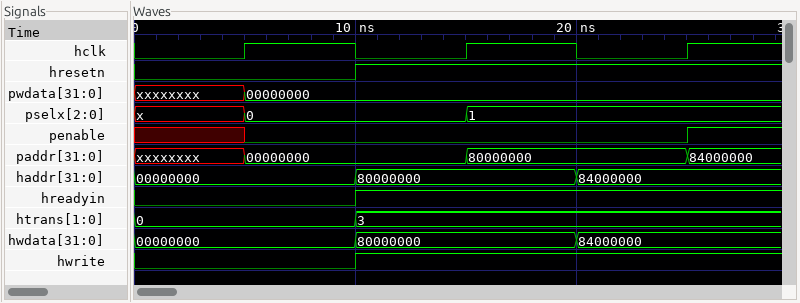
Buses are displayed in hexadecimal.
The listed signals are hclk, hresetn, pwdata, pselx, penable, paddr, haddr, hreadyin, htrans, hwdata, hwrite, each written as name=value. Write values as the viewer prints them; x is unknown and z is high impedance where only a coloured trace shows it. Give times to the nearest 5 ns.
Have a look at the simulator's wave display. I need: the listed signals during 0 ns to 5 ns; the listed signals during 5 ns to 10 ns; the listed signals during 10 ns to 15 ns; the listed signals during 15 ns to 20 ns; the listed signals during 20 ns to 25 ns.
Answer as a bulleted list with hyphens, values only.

- hclk=0, hresetn=0, pwdata=xxxxxxxx, pselx=x, penable=x, paddr=xxxxxxxx, haddr=00000000, hreadyin=0, htrans=0, hwdata=00000000, hwrite=0
- hclk=1, hresetn=0, pwdata=00000000, pselx=0, penable=0, paddr=00000000, haddr=00000000, hreadyin=0, htrans=0, hwdata=00000000, hwrite=0
- hclk=0, hresetn=1, pwdata=00000000, pselx=0, penable=0, paddr=00000000, haddr=80000000, hreadyin=1, htrans=3, hwdata=80000000, hwrite=1
- hclk=1, hresetn=1, pwdata=00000000, pselx=1, penable=0, paddr=80000000, haddr=80000000, hreadyin=1, htrans=3, hwdata=80000000, hwrite=1
- hclk=0, hresetn=1, pwdata=00000000, pselx=1, penable=0, paddr=80000000, haddr=84000000, hreadyin=1, htrans=3, hwdata=84000000, hwrite=1
